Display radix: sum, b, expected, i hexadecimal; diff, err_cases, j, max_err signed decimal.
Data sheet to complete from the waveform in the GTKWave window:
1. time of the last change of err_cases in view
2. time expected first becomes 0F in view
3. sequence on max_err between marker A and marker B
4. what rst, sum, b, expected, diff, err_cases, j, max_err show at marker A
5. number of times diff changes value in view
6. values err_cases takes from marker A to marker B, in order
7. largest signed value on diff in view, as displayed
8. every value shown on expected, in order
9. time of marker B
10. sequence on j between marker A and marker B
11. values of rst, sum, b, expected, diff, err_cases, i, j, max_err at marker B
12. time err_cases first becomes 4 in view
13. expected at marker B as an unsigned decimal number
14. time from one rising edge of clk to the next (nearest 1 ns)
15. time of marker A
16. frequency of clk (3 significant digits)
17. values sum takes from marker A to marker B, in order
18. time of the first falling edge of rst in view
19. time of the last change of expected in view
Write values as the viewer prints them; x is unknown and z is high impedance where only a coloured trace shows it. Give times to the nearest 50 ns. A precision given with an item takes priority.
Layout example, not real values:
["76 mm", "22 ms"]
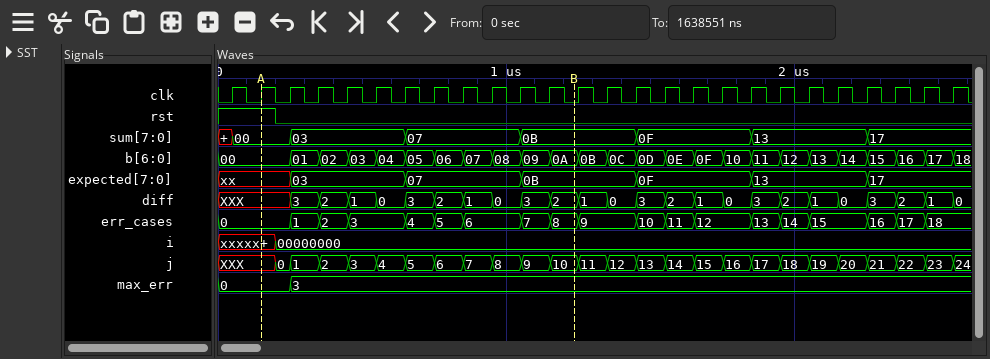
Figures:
["2450 ns", "1450 ns", "0, 3", "rst=1, sum=00, b=00, expected=xx, diff=XXX, err_cases=0, j=XXX, max_err=0", "24", "0, 1, 2, 3, 4, 5, 6, 7, 8", "3", "xx, 03, 07, 0B, 0F, 13, 17", "1250 ns", "XXX, 0, 1, 2, 3, 4, 5, 6, 7, 8, 9, 10", "rst=0, sum=0B, b=0A, expected=0B, diff=2, err_cases=8, i=00000000, j=10, max_err=3", "650 ns", "11", "100 ns", "150 ns", "10.0 MHz", "00, 03, 07, 0B", "200 ns", "2250 ns"]
